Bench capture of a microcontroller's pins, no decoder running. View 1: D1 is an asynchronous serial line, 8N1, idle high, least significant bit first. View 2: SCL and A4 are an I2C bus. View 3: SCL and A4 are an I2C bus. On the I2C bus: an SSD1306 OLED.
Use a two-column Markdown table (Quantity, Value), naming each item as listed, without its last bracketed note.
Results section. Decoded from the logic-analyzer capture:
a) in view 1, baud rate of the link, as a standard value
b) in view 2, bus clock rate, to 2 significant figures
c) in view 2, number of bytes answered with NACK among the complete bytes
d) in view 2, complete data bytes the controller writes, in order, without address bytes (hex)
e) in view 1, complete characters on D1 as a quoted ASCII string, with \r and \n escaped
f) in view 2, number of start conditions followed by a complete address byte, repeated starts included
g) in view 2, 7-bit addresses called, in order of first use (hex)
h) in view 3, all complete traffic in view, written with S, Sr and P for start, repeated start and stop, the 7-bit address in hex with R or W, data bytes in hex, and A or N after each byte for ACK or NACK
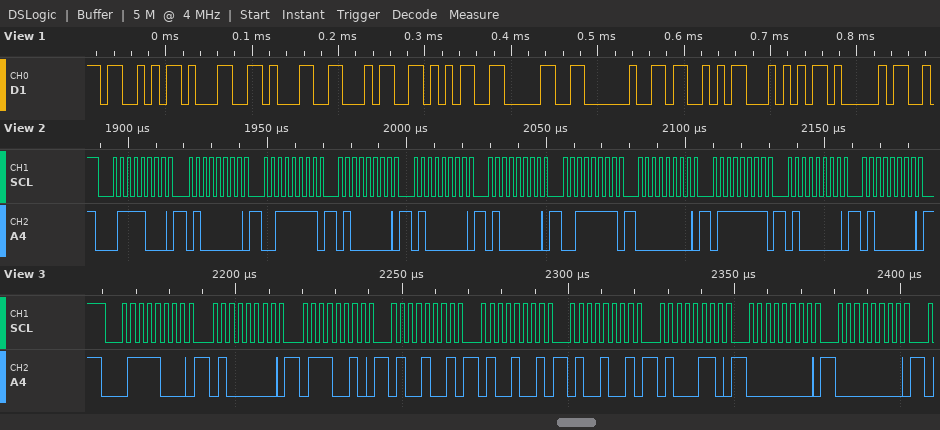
| Quantity | Value |
|---|---|
| in view 1, baud rate of the link, as a standard value | 115200 baud |
| in view 2, bus clock rate, to 2 significant figures | 400 kHz |
| in view 2, number of bytes answered with NACK among the complete bytes | 0 |
| in view 2, complete data bytes the controller writes, in order, without address bytes | 40 3F 40 40 40 3F 00 7F 40 40 |
| in view 1, complete characters on D1 as a quoted ASCII string, with \r and \n escaped | "S11450 STA" |
| in view 2, number of start conditions followed by a complete address byte, repeated starts included | 1 |
| in view 2, 7-bit addresses called, in order of first use | 0x3C |
| in view 3, all complete traffic in view, written with S, Sr and P for start, repeated start and stop, the 7-bit address in hex with R or W, data bytes in hex, and A or N after each byte for ACK or NACK | S 3CW A 40 A 72 A 49 A 49 A 49 A 46 A 00 A 00 A |
